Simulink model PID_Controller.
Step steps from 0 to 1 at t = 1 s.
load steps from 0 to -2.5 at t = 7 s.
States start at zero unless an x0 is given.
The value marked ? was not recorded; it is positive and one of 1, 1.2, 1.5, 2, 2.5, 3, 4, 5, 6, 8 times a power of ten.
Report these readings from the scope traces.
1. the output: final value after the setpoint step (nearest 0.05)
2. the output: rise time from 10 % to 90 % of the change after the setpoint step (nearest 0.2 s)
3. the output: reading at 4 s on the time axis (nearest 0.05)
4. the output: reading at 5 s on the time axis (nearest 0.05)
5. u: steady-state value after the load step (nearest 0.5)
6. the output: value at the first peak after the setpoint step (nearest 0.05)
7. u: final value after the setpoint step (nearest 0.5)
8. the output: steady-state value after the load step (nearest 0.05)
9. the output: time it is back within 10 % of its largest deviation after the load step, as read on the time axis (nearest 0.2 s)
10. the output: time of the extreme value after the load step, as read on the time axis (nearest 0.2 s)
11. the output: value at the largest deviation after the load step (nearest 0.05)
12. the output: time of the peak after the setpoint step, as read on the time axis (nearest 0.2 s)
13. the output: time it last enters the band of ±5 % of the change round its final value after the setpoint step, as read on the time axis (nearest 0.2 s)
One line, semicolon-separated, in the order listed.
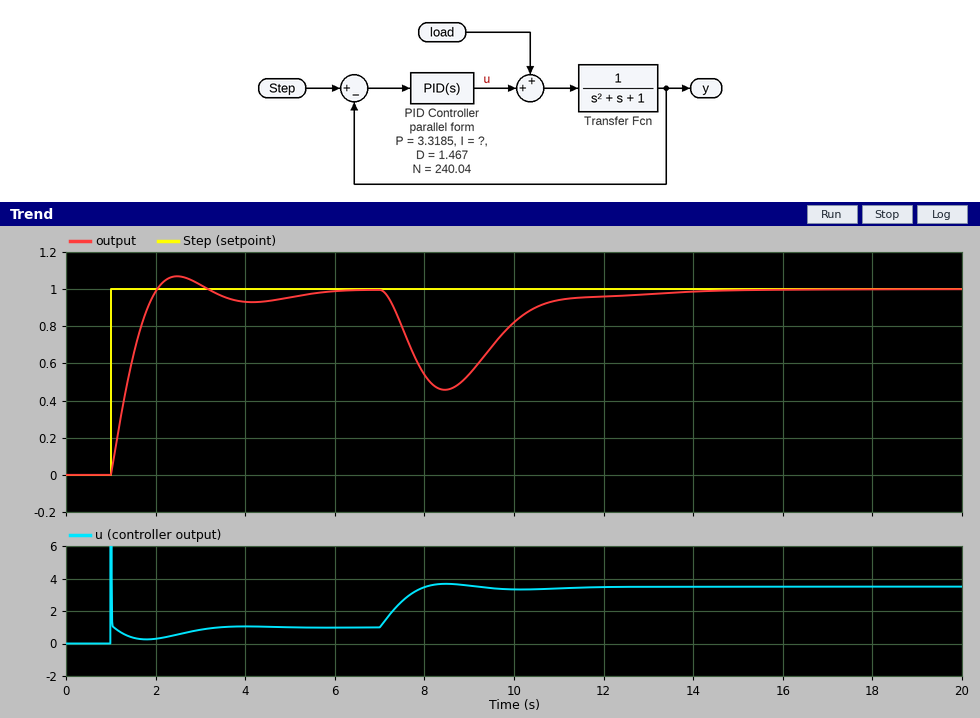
1.00; 0.8 s; 0.95; 0.95; 3.5; 1.05; 1.0; 1.00; 11.2 s; 8.4 s; 0.45; 2.4 s; 4.8 s
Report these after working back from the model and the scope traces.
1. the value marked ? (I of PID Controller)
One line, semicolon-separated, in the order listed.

2
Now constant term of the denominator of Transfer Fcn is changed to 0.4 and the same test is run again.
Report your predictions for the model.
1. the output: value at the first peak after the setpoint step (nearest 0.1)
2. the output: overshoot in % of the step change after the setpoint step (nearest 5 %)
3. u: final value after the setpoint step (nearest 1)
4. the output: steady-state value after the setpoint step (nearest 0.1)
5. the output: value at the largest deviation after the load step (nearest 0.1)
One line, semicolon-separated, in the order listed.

1.2; 20 %; 0; 1.0; 0.4
